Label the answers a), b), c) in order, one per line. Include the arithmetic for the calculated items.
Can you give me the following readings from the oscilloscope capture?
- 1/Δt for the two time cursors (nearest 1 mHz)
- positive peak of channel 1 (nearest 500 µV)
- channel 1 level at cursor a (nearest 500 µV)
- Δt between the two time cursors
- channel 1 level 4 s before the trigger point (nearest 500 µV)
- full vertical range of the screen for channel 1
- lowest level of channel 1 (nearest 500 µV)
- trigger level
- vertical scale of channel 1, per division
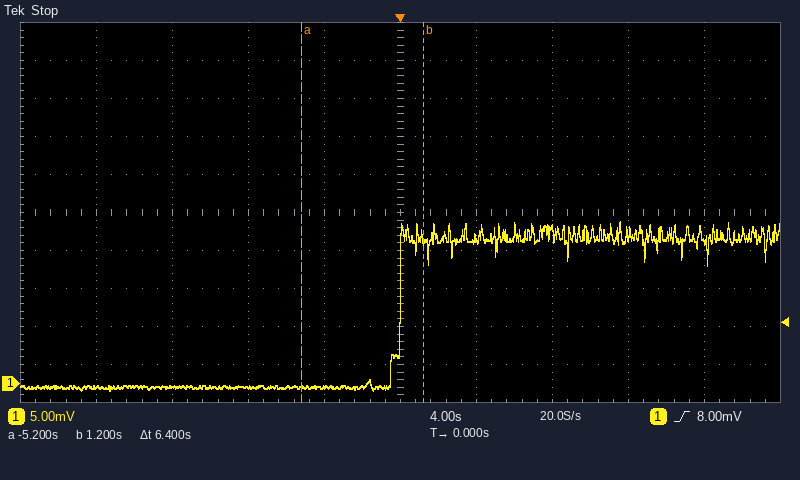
a) 1 / 6.4 s ≈ 156 mHz
b) 21.5 mV
c) -500 µV
d) 6.4 s
e) -500 µV
f) 50 mV
g) -1.0 mV
h) 8.00 mV
i) 5 mV
